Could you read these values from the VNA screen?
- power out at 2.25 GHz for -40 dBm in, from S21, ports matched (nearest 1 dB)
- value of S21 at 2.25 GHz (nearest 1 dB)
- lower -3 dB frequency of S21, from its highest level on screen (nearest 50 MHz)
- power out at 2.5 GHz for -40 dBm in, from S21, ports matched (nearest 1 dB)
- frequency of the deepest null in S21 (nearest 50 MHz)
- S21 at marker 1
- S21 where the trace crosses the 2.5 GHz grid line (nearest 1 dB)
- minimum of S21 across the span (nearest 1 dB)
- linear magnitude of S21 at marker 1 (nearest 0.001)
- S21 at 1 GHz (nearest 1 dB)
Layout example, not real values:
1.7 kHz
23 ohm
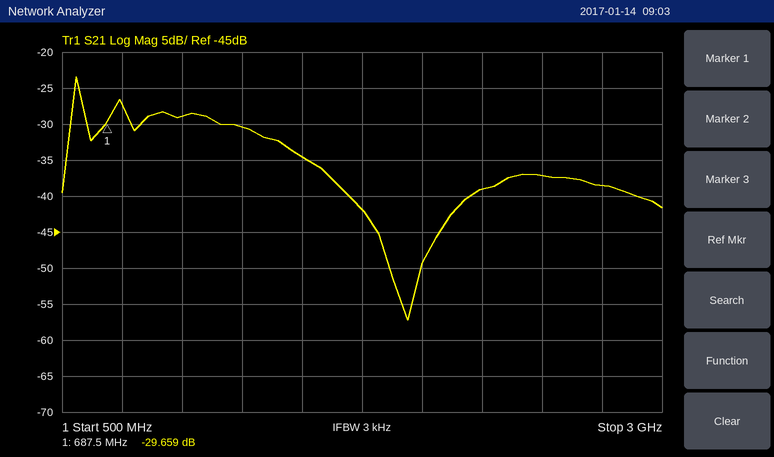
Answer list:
-79 dBm
-39 dB
550 MHz
-77 dBm
1.95 GHz
-29.659 dB
-37 dB
-57 dB
0.033
-29 dB
